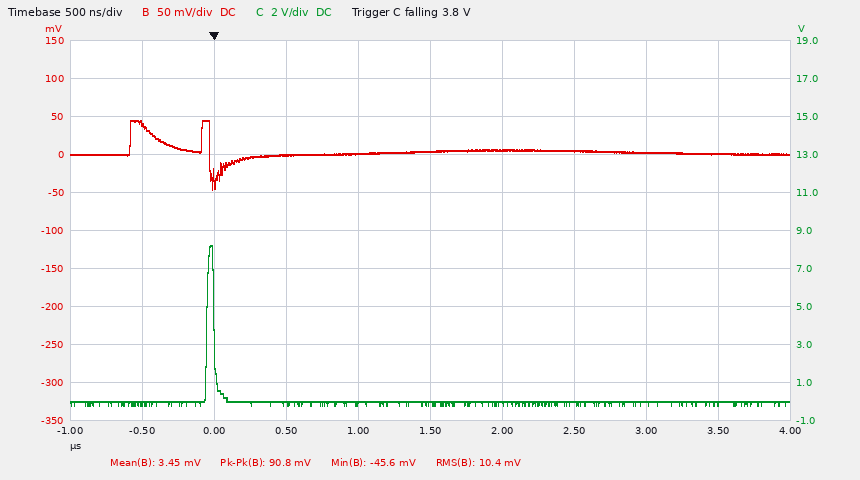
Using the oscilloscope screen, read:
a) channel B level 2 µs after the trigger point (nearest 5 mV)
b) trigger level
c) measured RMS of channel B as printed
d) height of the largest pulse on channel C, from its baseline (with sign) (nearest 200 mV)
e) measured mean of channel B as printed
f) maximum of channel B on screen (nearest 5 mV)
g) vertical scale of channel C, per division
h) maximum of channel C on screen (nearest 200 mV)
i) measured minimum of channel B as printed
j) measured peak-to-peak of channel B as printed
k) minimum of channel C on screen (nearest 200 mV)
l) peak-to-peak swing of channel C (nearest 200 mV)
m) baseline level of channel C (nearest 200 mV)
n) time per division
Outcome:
5 mV
3.8 V
10.4 mV
+8.2 V
3.45 mV
45 mV
2 V
8.2 V
-45.6 mV
90.8 mV
-200 mV
8.4 V
0.0 V
500 ns
